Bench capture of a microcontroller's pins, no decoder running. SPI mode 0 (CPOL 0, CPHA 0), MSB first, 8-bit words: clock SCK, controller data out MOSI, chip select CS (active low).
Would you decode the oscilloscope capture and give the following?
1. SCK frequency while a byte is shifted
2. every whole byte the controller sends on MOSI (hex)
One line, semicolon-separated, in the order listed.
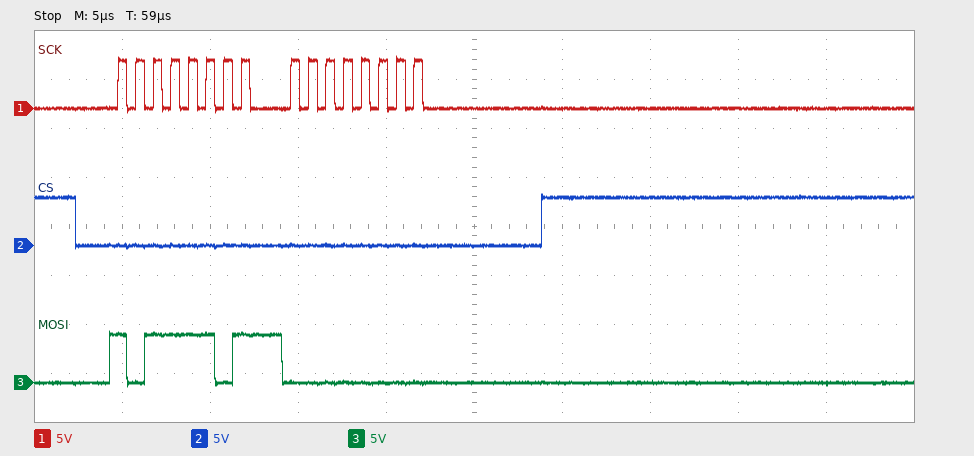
1 MHz; BD 00
